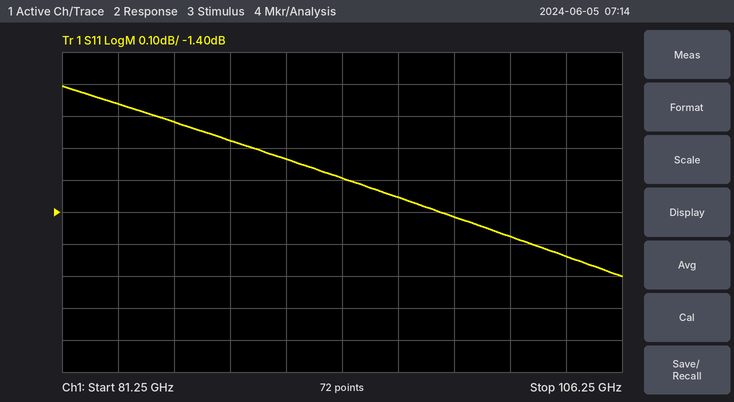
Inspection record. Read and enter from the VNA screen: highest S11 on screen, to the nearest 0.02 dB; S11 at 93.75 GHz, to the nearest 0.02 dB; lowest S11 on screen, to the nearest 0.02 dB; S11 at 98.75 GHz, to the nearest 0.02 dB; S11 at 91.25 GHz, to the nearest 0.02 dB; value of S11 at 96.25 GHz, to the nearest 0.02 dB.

-1.00 dB
-1.30 dB
-1.60 dB
-1.42 dB
-1.24 dB
-1.36 dB
